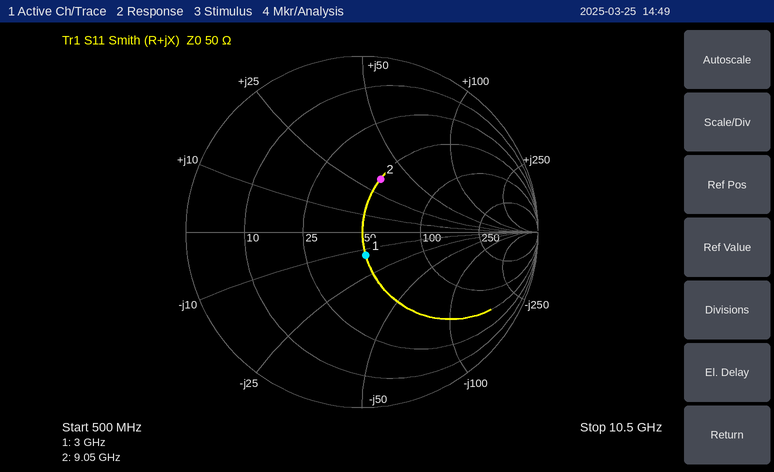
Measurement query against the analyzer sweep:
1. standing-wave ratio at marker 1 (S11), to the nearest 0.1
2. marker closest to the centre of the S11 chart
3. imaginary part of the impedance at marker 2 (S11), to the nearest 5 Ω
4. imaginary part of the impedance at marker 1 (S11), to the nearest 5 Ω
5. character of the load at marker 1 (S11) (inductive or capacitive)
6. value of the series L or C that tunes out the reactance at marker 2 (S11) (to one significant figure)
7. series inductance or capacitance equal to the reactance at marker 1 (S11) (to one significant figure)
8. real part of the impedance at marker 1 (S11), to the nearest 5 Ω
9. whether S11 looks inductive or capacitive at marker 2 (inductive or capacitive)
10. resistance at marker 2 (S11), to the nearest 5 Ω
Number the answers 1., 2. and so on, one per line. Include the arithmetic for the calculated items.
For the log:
1. 1.3
2. marker 1
3. +35 Ω
4. -15 Ω
5. capacitive
6. C = 1/(2π × 9.05 GHz × 35 Ω) ≈ 502 fF, so 500 fF to one significant figure
7. C = 1/(2π × 3 GHz × 15 Ω) ≈ 4 pF
8. 50 Ω
9. inductive
10. 50 Ω
